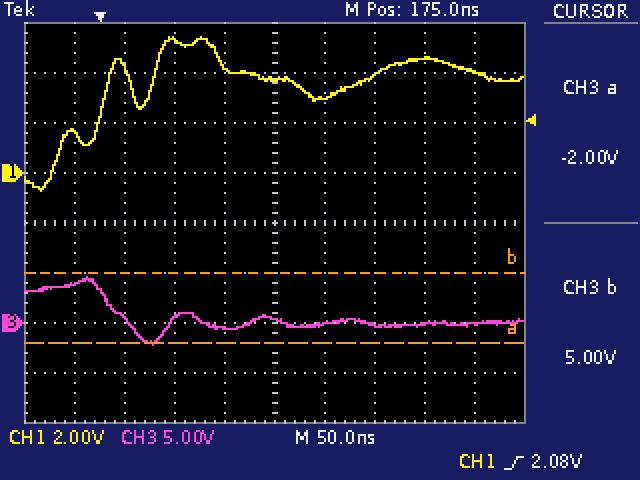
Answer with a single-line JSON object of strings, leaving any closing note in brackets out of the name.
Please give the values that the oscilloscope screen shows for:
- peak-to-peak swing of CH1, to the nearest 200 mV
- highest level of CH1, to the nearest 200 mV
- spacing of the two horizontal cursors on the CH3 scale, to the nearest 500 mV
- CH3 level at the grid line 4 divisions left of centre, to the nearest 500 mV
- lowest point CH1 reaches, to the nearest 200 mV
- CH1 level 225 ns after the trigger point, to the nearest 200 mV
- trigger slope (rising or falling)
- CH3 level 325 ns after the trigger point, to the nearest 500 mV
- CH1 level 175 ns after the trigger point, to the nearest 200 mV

{"peak-to-peak swing of CH1, to the nearest 200 mV": "6.2 V", "highest level of CH1, to the nearest 200 mV": "5.4 V", "spacing of the two horizontal cursors on the CH3 scale, to the nearest 500 mV": "7.0 V", "CH3 level at the grid line 4 divisions left of centre, to the nearest 500 mV": "4.0 V", "lowest point CH1 reaches, to the nearest 200 mV": "-800 mV", "CH1 level 225 ns after the trigger point, to the nearest 200 mV": "3.0 V", "trigger slope": "rising", "CH3 level 325 ns after the trigger point, to the nearest 500 mV": "0.0 V", "CH1 level 175 ns after the trigger point, to the nearest 200 mV": "3.8 V"}
